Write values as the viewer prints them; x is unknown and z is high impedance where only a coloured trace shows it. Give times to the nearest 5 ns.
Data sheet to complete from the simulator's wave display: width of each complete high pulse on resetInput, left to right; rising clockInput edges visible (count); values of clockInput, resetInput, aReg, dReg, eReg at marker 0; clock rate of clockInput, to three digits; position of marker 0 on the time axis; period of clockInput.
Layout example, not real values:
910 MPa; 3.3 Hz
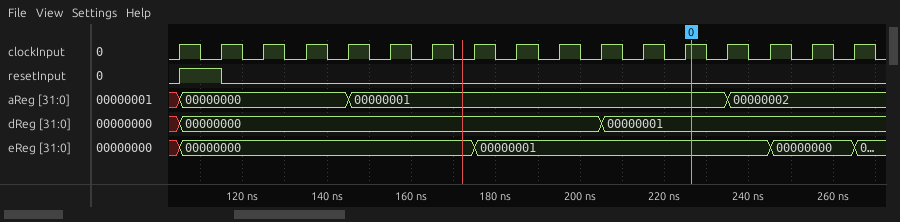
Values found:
10 ns; 17; clockInput=1, resetInput=0, aReg=00000001, dReg=00000001, eReg=00000001; 100 MHz; 225 ns; 10 ns
